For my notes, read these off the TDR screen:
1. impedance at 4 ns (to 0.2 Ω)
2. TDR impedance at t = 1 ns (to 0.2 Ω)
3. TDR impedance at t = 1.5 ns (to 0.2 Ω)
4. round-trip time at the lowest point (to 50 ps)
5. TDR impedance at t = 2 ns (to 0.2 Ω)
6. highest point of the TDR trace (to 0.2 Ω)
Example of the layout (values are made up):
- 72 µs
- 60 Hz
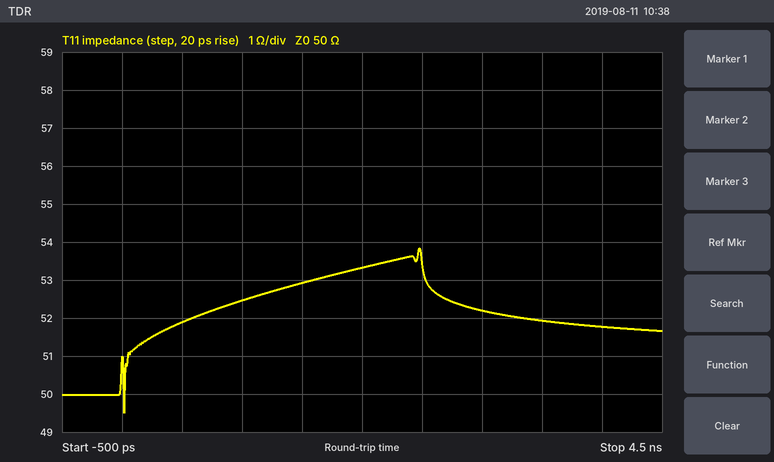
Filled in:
- 51.8 Ω
- 52.4 Ω
- 53.0 Ω
- 0 ps
- 53.4 Ω
- 53.8 Ω
